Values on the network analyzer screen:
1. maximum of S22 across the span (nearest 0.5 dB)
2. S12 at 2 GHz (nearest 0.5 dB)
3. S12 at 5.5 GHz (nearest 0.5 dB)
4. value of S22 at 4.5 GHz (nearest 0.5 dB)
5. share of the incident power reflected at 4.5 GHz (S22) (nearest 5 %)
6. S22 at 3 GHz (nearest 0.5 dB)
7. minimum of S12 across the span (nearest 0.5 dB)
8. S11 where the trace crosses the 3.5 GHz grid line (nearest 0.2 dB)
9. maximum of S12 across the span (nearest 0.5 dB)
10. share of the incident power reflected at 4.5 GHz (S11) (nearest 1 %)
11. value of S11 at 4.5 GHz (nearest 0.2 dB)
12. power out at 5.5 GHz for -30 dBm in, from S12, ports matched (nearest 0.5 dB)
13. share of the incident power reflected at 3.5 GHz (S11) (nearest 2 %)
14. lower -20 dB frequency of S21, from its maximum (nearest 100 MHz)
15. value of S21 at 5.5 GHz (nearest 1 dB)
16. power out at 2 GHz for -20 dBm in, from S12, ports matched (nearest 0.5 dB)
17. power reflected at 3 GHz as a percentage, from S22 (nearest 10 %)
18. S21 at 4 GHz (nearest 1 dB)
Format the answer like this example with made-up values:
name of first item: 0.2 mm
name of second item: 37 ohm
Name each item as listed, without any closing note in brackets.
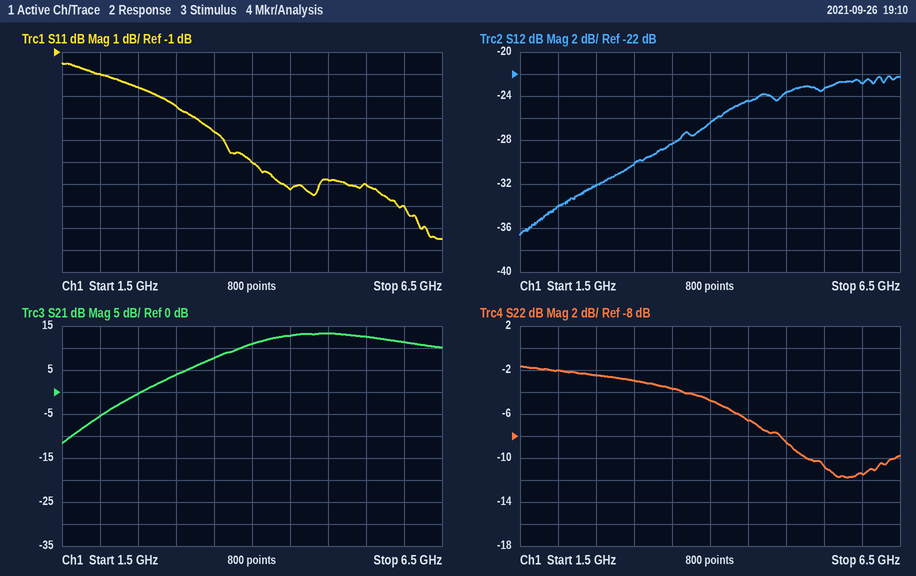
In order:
maximum of S22 across the span: -1.5 dB
S12 at 2 GHz: -34.0 dB
S12 at 5.5 GHz: -23.5 dB
value of S22 at 4.5 GHz: -6.5 dB
share of the incident power reflected at 4.5 GHz (S22): 20 %
S22 at 3 GHz: -3.0 dB
minimum of S12 across the span: -36.5 dB
S11 where the trace crosses the 3.5 GHz grid line: -4.6 dB
maximum of S12 across the span: -22.0 dB
share of the incident power reflected at 4.5 GHz (S11): 19 %
value of S11 at 4.5 GHz: -7.2 dB
power out at 5.5 GHz for -30 dBm in, from S12, ports matched: -53.5 dBm
share of the incident power reflected at 3.5 GHz (S11): 34 %
lower -20 dB frequency of S21, from its maximum: 1.9 GHz
value of S21 at 5.5 GHz: 13 dB
power out at 2 GHz for -20 dBm in, from S12, ports matched: -54.0 dBm
power reflected at 3 GHz as a percentage, from S22: 50 %
S21 at 4 GHz: 11 dB
